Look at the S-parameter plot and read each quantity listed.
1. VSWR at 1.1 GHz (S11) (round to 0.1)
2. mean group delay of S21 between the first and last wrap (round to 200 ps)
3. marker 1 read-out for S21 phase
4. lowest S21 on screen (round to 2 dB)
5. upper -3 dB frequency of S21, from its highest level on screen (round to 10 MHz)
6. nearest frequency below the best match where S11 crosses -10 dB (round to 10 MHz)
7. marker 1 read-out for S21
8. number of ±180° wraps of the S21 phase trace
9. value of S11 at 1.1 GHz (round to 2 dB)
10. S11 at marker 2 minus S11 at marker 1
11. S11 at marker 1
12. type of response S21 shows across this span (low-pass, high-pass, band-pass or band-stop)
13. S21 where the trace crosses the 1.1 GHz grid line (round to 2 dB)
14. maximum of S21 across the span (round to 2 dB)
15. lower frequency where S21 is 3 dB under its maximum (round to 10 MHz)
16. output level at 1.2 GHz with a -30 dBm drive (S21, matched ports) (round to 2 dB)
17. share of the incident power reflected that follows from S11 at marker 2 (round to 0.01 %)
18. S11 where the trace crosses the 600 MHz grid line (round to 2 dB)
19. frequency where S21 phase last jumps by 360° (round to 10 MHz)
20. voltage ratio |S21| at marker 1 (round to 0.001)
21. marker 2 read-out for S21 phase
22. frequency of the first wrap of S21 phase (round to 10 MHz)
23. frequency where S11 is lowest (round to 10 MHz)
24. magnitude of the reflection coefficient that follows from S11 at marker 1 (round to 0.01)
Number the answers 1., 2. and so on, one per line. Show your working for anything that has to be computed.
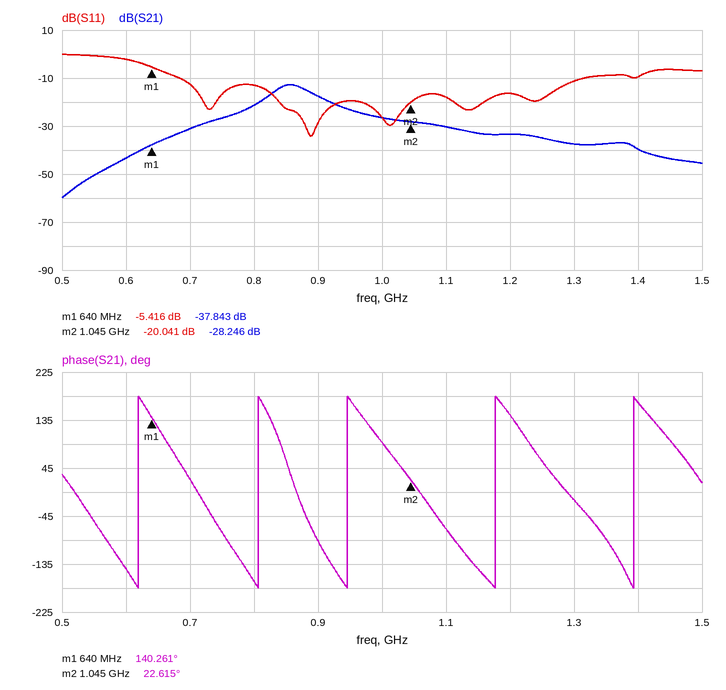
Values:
1. |Γ| = 10^(-18/20) = 0.1259; VSWR = (1 + 0.1259)/(1 − 0.1259) ≈ 1.3
2. 4 cycles / (1.39 GHz − 620 MHz) ≈ 5.2 ns
3. 140.261°
4. -60 dB
5. 890 MHz
6. 680 MHz
7. -37.843 dB
8. 5
9. -18 dB
10. -20.041 − (-5.416) = -14.625 dB
11. -5.416 dB
12. band-pass
13. -30 dB
14. -12 dB
15. 830 MHz
16. -30 dBm + (-34 dB) = -64 dBm
17. 10^(-20.041/10) ≈ 0.99 %
18. -2 dB
19. 1.39 GHz
20. 10^(-37.843/20) ≈ 0.013
21. 22.615°
22. 620 MHz
23. 890 MHz
24. 10^(-5.416/20) ≈ 0.54
